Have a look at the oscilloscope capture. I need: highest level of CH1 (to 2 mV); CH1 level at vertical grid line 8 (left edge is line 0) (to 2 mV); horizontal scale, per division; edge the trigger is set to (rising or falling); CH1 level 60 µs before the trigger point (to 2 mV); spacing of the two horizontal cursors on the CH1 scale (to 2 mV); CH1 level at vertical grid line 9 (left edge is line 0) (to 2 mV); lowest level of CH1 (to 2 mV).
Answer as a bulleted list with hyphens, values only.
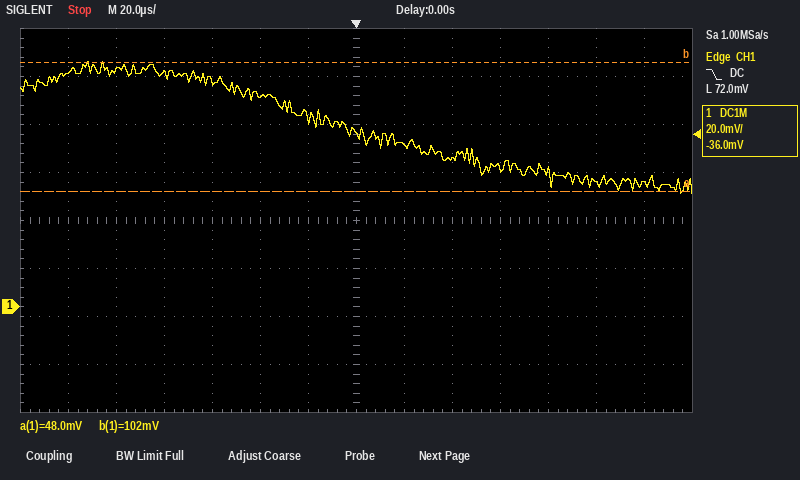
- 102 mV
- 68 mV
- 20 µs
- falling
- 94 mV
- 54 mV
- 62 mV
- 48 mV
